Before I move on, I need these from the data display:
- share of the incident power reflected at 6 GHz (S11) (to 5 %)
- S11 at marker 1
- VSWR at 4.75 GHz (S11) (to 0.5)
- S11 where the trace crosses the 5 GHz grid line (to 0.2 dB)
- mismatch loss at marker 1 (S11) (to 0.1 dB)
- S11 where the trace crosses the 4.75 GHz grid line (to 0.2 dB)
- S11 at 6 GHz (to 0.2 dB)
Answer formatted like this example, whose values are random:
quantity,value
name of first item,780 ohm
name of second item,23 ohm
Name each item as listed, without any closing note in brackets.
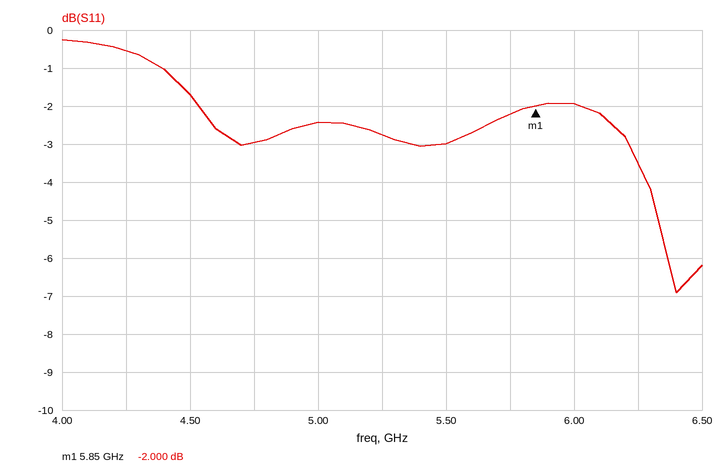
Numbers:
quantity,value
share of the incident power reflected at 6 GHz (S11),65 %
S11 at marker 1,-2.000 dB
VSWR at 4.75 GHz (S11),6.0
S11 where the trace crosses the 5 GHz grid line,-2.4 dB
mismatch loss at marker 1 (S11),4.3 dB
S11 where the trace crosses the 4.75 GHz grid line,-3.0 dB
S11 at 6 GHz,-2.0 dB
